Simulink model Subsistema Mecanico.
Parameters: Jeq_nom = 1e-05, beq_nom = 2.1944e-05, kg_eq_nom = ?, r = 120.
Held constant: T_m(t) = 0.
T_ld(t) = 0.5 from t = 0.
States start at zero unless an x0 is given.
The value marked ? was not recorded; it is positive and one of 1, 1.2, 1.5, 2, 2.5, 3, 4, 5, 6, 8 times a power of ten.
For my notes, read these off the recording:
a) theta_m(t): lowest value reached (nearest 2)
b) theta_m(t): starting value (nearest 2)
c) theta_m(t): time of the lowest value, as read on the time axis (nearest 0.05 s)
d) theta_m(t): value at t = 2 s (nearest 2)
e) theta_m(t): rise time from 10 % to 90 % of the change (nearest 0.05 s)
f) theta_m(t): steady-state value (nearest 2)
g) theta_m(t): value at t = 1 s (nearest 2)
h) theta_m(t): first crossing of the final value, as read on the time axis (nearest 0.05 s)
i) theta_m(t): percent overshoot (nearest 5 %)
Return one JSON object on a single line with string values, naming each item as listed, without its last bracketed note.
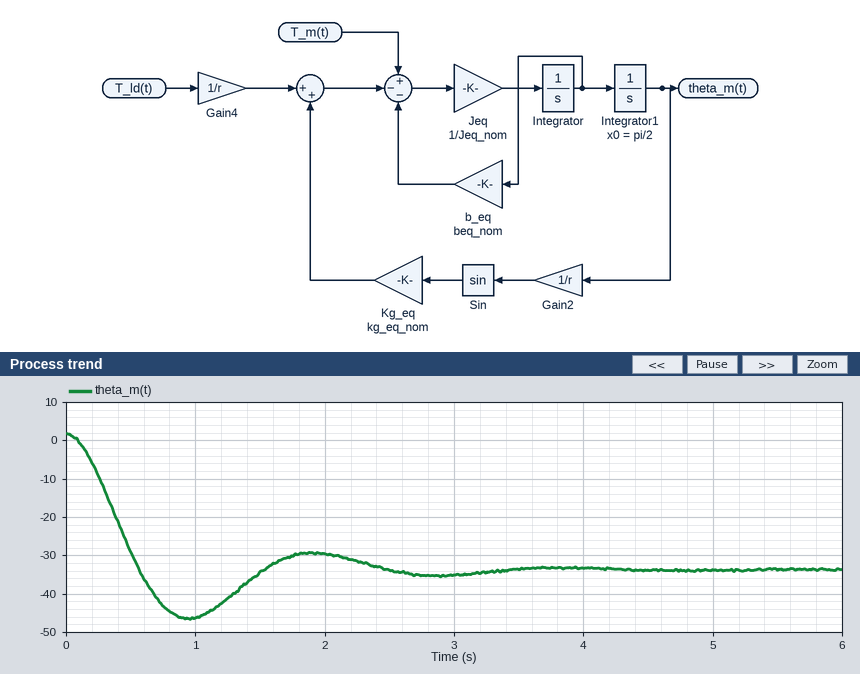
{"theta_m(t): lowest value reached": "-46", "theta_m(t): starting value": "2", "theta_m(t): time of the lowest value, as read on the time axis": "0.95 s", "theta_m(t): value at t = 2 s": "-30", "theta_m(t): rise time from 10 % to 90 % of the change": "0.40 s", "theta_m(t): steady-state value": "-34", "theta_m(t): value at t = 1 s": "-46", "theta_m(t): first crossing of the final value, as read on the time axis": "0.55 s", "theta_m(t): percent overshoot": "35 %"}
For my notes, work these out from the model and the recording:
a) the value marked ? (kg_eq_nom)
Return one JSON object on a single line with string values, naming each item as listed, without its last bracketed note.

{"the value marked ?": "0.015"}
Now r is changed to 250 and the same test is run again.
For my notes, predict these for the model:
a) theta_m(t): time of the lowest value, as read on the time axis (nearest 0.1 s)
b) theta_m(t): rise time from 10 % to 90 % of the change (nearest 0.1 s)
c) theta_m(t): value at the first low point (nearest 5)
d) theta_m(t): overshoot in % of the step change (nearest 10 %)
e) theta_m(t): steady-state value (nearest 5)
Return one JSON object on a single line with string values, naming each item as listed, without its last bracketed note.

{"theta_m(t): time of the lowest value, as read on the time axis": "1.4 s", "theta_m(t): rise time from 10 % to 90 % of the change": "0.6 s", "theta_m(t): value at the first low point": "-40", "theta_m(t): overshoot in % of the step change": "20 %", "theta_m(t): steady-state value": "-35"}
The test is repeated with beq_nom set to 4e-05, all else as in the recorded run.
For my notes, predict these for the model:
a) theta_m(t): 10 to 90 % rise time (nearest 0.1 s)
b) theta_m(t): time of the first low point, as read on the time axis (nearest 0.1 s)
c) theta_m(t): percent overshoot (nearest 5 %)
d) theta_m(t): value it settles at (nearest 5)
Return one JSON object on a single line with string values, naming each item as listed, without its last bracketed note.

{"theta_m(t): 10 to 90 % rise time": "0.5 s", "theta_m(t): time of the first low point, as read on the time axis": "1.1 s", "theta_m(t): percent overshoot": "10 %", "theta_m(t): value it settles at": "-35"}
